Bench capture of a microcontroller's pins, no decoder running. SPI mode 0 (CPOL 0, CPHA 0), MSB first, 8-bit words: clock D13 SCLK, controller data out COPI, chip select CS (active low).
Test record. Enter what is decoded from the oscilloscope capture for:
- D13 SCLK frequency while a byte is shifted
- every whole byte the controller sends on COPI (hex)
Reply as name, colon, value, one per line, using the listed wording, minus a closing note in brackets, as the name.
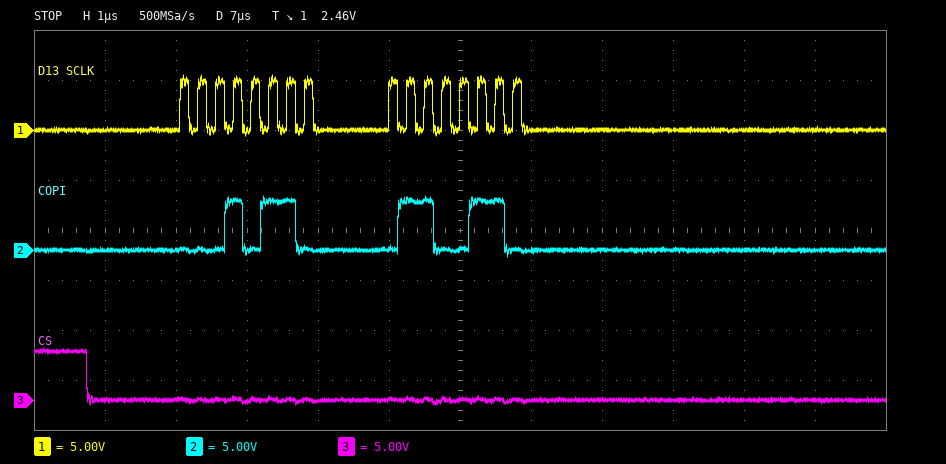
D13 SCLK frequency while a byte is shifted: 4 MHz
every whole byte the controller sends on COPI: 0x16 0x66
